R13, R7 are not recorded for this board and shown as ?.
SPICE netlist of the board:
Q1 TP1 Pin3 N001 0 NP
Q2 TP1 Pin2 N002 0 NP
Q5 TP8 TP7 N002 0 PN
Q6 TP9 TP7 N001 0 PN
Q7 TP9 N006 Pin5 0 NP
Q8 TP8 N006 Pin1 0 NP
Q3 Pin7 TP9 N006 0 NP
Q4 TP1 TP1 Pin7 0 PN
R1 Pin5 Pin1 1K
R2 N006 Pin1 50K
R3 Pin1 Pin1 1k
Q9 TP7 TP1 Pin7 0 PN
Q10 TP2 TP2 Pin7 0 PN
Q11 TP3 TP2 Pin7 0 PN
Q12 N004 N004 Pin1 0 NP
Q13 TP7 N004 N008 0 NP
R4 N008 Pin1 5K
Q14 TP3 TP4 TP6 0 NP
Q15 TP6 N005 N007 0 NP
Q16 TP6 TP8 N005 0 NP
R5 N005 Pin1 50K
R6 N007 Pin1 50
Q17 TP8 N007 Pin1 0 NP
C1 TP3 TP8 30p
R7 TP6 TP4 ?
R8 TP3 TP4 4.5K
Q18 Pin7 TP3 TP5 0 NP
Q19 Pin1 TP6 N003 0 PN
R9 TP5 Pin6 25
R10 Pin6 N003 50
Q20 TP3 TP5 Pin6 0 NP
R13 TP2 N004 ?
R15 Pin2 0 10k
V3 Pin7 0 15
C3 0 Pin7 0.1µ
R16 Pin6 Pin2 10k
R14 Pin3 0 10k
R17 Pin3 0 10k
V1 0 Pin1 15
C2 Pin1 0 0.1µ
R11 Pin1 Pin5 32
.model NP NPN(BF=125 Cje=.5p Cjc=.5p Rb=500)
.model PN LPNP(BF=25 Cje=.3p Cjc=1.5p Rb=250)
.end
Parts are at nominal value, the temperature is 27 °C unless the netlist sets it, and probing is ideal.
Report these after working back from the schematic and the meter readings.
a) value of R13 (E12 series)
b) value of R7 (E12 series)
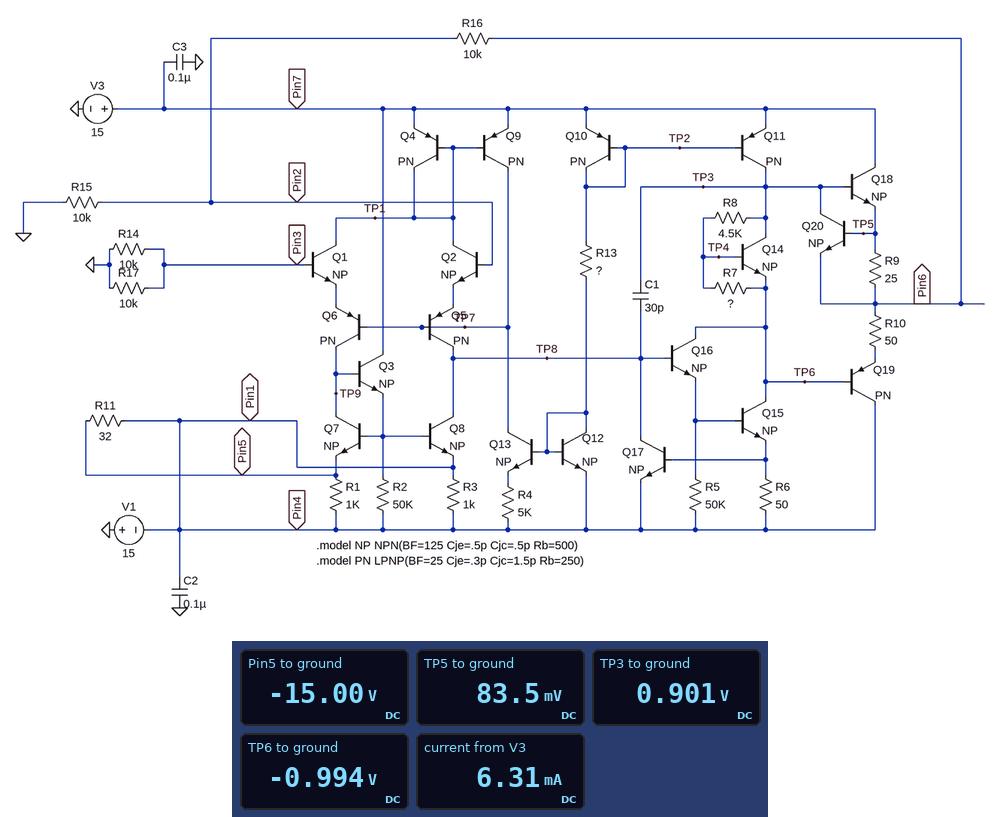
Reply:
18 kΩ
3.3 kΩ
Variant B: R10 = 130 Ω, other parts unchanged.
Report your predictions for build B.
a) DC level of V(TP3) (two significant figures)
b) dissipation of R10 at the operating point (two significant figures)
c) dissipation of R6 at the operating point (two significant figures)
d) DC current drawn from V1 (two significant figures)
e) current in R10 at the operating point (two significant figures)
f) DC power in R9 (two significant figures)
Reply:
850 mV
460 µW
110 µW
5.0 mA
1.9 mA
88 µW
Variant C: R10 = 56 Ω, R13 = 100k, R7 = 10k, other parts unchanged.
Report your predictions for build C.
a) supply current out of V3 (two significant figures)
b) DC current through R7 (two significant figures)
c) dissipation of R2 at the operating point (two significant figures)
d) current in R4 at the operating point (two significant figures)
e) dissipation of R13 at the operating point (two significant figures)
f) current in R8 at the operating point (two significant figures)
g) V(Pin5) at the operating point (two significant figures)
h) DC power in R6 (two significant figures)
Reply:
590 µA
73 µA
8.4 µW
15 µA
8.1 mW
75 µA
-15 V
3.1 µW
